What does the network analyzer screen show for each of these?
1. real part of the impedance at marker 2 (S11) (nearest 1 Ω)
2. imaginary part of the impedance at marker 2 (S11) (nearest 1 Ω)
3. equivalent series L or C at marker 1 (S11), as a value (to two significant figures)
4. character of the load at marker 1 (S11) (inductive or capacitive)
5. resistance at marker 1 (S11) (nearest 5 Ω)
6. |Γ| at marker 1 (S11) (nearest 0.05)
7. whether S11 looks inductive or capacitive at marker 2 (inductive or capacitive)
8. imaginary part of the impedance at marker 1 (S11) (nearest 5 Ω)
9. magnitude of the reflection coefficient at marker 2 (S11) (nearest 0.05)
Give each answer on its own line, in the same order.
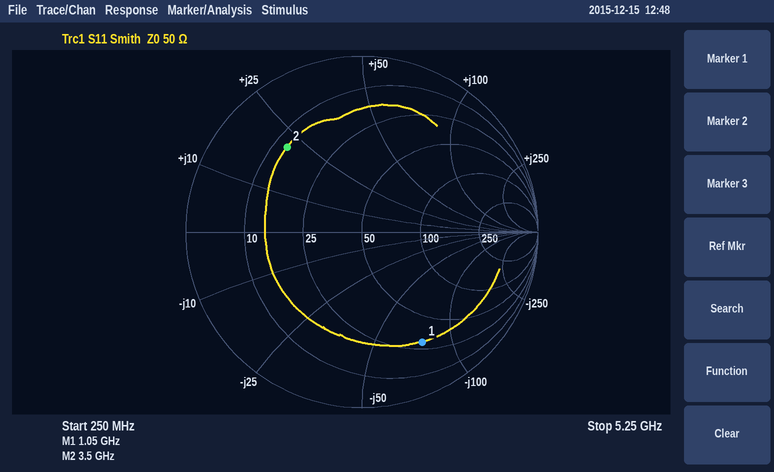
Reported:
13 Ω
+21 Ω
2.0 pF
capacitive
30 Ω
0.70
inductive
-75 Ω
0.65
